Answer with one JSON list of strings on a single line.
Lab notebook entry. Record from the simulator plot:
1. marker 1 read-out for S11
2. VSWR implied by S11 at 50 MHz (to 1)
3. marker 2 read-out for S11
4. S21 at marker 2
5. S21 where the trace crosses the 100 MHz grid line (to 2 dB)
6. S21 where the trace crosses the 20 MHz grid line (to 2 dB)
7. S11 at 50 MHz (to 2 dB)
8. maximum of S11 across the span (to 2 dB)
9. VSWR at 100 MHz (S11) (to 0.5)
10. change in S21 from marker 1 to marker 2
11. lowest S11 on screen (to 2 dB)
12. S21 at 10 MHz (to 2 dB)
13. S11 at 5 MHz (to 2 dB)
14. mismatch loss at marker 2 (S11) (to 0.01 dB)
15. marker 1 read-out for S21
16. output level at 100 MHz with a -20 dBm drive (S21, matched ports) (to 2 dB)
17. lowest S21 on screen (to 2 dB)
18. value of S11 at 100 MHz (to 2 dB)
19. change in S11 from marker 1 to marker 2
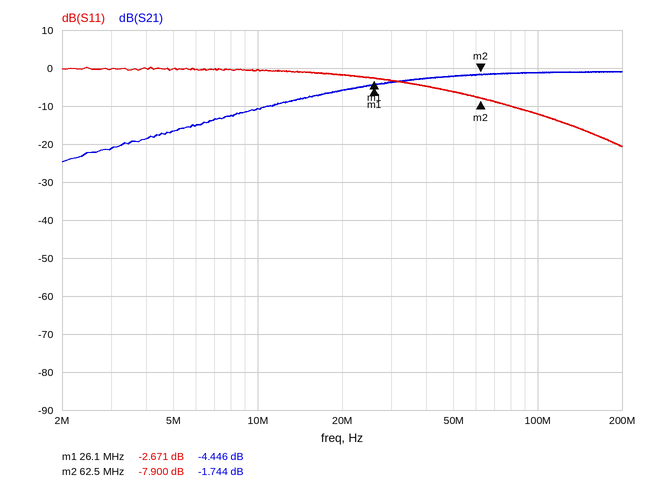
["-2.671 dB", "3", "-7.900 dB", "-1.744 dB", "-2 dB", "-6 dB", "-6 dB", "0 dB", "1.5", "2.702 dB", "-20 dB", "-10 dB", "0 dB", "0.77 dB", "-4.446 dB", "-22 dBm", "-24 dB", "-12 dB", "-5.229 dB"]
